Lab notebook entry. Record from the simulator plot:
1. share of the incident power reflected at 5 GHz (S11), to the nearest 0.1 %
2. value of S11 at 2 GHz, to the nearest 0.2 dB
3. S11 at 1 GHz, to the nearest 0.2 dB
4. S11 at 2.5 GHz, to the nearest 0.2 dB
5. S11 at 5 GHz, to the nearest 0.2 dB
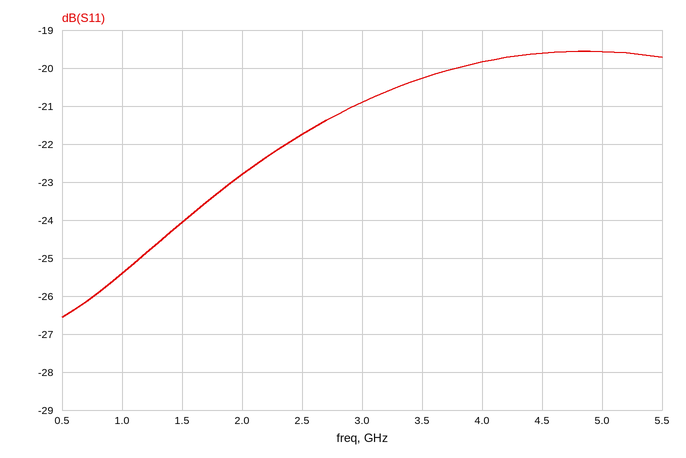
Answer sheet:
1.1 %
-22.8 dB
-25.4 dB
-21.8 dB
-19.6 dB
